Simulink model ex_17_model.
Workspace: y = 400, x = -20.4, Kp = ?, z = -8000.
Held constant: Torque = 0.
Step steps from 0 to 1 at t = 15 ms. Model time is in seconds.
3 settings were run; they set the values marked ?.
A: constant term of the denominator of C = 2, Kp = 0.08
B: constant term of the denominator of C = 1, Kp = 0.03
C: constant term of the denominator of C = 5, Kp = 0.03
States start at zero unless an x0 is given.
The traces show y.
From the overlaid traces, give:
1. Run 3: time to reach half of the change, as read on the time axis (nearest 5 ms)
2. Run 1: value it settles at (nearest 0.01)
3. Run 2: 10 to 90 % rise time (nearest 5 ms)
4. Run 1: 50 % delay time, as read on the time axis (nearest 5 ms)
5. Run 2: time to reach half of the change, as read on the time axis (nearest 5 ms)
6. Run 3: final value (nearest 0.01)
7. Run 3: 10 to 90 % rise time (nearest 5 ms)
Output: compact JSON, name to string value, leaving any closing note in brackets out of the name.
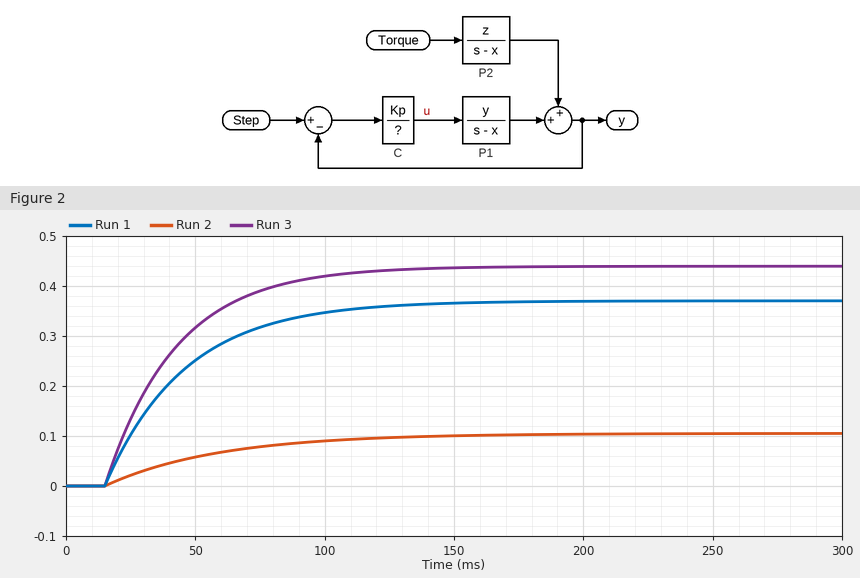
{"Run 3: time to reach half of the change, as read on the time axis": "35 ms", "Run 1: value it settles at": "0.37", "Run 2: 10 to 90 % rise time": "95 ms", "Run 1: 50 % delay time, as read on the time axis": "35 ms", "Run 2: time to reach half of the change, as read on the time axis": "45 ms", "Run 3: final value": "0.44", "Run 3: 10 to 90 % rise time": "60 ms"}
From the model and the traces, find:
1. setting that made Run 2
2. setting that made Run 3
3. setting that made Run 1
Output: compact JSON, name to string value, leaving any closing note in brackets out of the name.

{"setting that made Run 2": "C", "setting that made Run 3": "A", "setting that made Run 1": "B"}
